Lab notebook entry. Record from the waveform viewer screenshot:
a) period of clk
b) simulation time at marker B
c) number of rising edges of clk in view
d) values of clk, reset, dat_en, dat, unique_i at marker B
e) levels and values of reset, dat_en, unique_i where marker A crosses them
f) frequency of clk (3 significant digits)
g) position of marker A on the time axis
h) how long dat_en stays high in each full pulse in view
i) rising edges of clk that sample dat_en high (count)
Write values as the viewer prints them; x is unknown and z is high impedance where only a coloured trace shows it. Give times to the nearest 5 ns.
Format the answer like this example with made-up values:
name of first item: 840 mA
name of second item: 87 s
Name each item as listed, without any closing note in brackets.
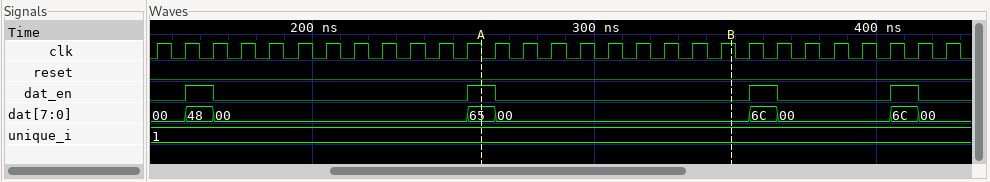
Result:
period of clk: 10 ns
simulation time at marker B: 350 ns
number of rising edges of clk in view: 29
values of clk, reset, dat_en, dat, unique_i at marker B: clk=1, reset=0, dat_en=0, dat=00, unique_i=1
levels and values of reset, dat_en, unique_i where marker A crosses them: reset=0, dat_en=1, unique_i=1
frequency of clk: 100 MHz
position of marker A on the time axis: 260 ns
how long dat_en stays high in each full pulse in view: 10 ns, 10 ns, 10 ns, 10 ns
rising edges of clk that sample dat_en high: 4
